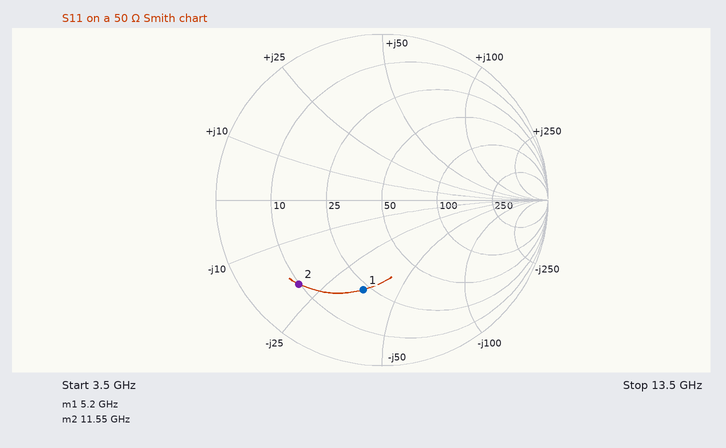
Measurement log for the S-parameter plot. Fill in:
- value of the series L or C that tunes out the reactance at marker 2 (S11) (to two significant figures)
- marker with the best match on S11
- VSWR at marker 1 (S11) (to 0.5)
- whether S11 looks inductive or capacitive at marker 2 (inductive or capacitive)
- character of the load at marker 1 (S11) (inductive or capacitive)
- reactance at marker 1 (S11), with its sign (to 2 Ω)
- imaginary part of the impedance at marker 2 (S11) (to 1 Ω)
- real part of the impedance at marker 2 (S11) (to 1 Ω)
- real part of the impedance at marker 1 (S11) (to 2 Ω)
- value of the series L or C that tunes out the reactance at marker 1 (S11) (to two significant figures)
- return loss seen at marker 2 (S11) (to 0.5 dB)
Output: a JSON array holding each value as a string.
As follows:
["280 pH", "marker 1", "3.5", "capacitive", "capacitive", "-36 Ω", "-20 Ω", "10 Ω", "22 Ω", "1.1 nH", "3.0 dB"]
